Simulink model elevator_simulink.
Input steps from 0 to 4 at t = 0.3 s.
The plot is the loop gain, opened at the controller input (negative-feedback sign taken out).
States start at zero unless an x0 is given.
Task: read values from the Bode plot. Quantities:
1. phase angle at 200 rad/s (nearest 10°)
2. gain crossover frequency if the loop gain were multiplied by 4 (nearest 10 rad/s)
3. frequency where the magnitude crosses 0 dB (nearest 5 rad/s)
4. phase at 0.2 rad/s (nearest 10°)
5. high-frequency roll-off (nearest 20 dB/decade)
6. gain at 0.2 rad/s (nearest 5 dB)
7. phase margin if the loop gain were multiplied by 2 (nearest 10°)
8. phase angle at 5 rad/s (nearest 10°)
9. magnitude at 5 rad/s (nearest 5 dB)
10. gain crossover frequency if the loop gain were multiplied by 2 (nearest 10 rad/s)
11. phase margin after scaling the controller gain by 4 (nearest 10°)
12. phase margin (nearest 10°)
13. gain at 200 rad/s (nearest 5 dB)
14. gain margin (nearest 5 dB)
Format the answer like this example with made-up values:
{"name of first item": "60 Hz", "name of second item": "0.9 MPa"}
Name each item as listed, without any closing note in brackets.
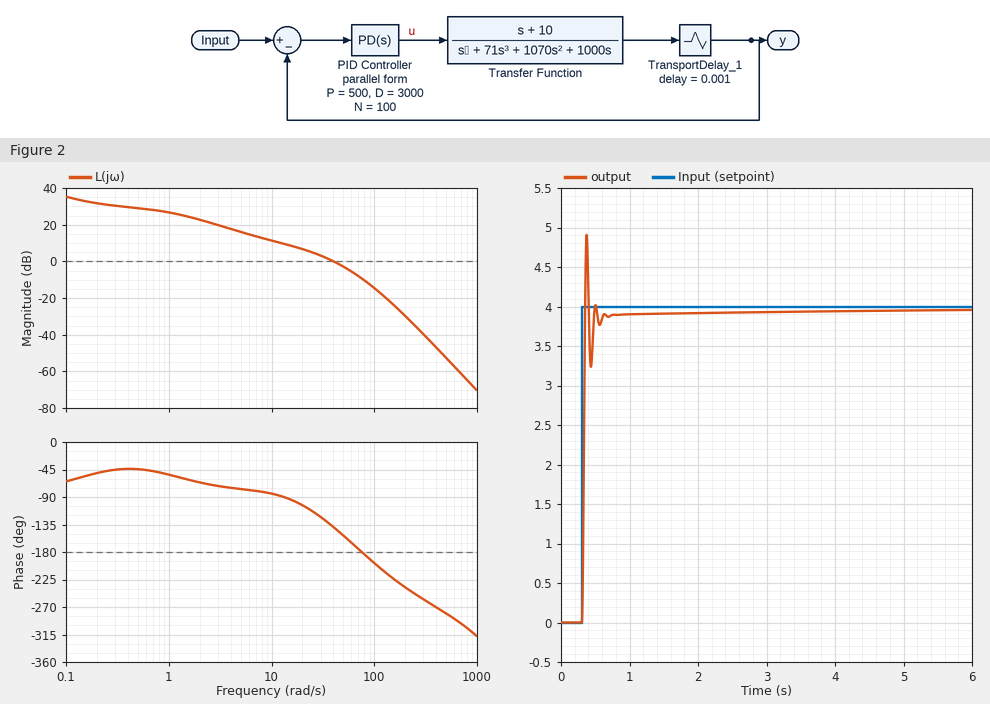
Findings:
{"phase angle at 200 rad/s": "-240°", "gain crossover frequency if the loop gain were multiplied by 4": "90 rad/s", "frequency where the magnitude crosses 0 dB": "40 rad/s", "phase at 0.2 rad/s": "-50°", "high-frequency roll-off": "-60 dB/decade", "gain at 0.2 rad/s": "30 dB", "phase margin if the loop gain were multiplied by 2": "10°", "phase angle at 5 rad/s": "-80°", "magnitude at 5 rad/s": "15 dB", "gain crossover frequency if the loop gain were multiplied by 2": "60 rad/s", "phase margin after scaling the controller gain by 4": "-10°", "phase margin": "40°", "gain at 200 rad/s": "-30 dB", "gain margin": "10 dB"}
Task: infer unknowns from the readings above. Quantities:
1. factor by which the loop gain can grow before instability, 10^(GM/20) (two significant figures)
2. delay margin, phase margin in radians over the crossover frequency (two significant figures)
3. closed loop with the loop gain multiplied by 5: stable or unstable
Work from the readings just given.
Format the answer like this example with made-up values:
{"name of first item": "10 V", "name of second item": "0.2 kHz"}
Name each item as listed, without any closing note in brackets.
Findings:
{"factor by which the loop gain can grow before instability, 10^(GM/20)": "3.2", "delay margin, phase margin in radians over the crossover frequency": "0.017 s", "closed loop with the loop gain multiplied by 5: stable or unstable": "unstable"}
